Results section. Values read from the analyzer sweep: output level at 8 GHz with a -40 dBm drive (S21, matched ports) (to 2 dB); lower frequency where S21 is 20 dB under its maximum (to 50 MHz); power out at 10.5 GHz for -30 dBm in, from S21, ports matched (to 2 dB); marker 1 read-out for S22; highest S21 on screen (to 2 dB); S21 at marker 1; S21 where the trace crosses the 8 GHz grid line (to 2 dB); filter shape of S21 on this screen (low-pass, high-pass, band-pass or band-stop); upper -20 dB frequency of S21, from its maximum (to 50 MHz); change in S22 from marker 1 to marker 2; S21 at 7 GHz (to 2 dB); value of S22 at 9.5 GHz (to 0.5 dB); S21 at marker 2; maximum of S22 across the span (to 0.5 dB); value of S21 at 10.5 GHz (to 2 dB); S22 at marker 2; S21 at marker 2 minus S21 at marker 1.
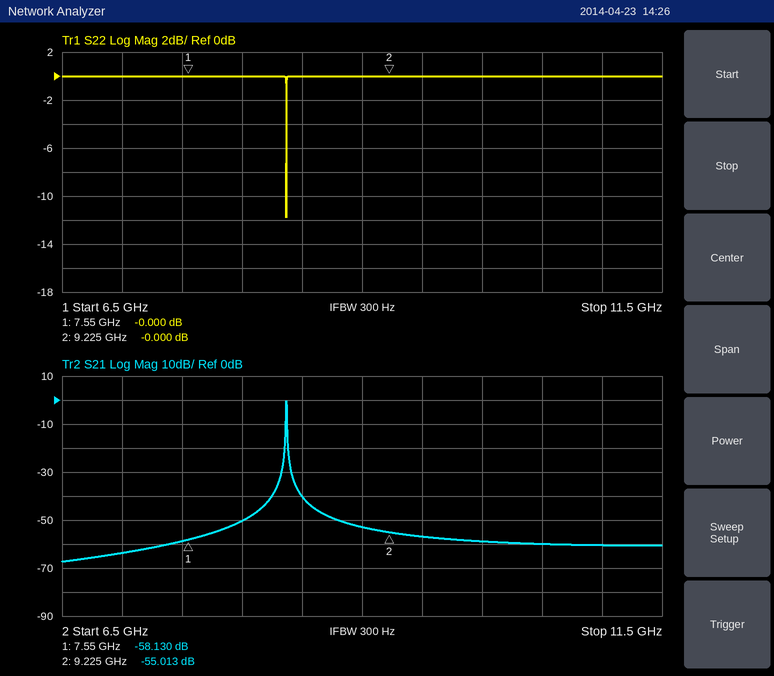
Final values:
-90 dBm
8.35 GHz
-90 dBm
-0.000 dB
0 dB
-58.130 dB
-50 dB
band-pass
8.40 GHz
0.000 dB
-64 dB
0.0 dB
-55.013 dB
0.0 dB
-60 dB
-0.000 dB
3.117 dB
